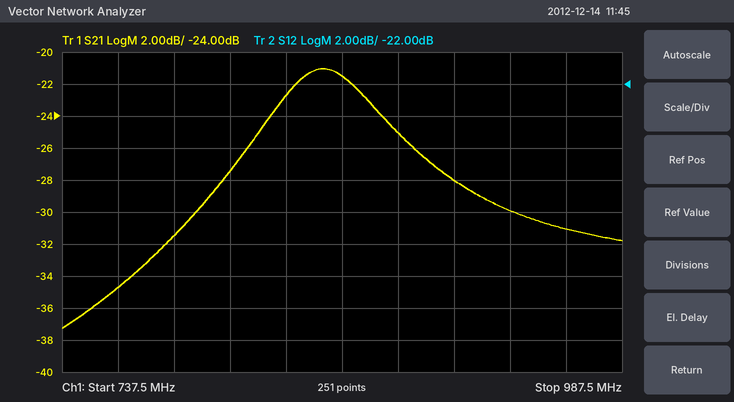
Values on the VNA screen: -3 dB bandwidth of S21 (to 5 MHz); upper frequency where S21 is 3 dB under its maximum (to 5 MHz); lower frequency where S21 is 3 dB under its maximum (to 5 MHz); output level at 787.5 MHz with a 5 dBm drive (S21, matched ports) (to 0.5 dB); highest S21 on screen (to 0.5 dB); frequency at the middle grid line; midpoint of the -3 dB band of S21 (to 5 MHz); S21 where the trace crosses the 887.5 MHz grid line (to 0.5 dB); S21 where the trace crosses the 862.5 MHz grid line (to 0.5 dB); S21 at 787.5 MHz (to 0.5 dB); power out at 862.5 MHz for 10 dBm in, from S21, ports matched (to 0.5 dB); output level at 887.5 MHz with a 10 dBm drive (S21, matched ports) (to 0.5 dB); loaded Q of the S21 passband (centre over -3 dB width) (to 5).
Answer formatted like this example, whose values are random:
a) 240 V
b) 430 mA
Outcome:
a) 50 MHz
b) 880 MHz
c) 830 MHz
d) -26.5 dBm
e) -21.0 dB
f) 862.5 MHz
g) 855 MHz
h) -25.0 dB
i) -21.5 dB
j) -31.5 dB
k) -11.5 dBm
l) -15.0 dBm
m) 15
